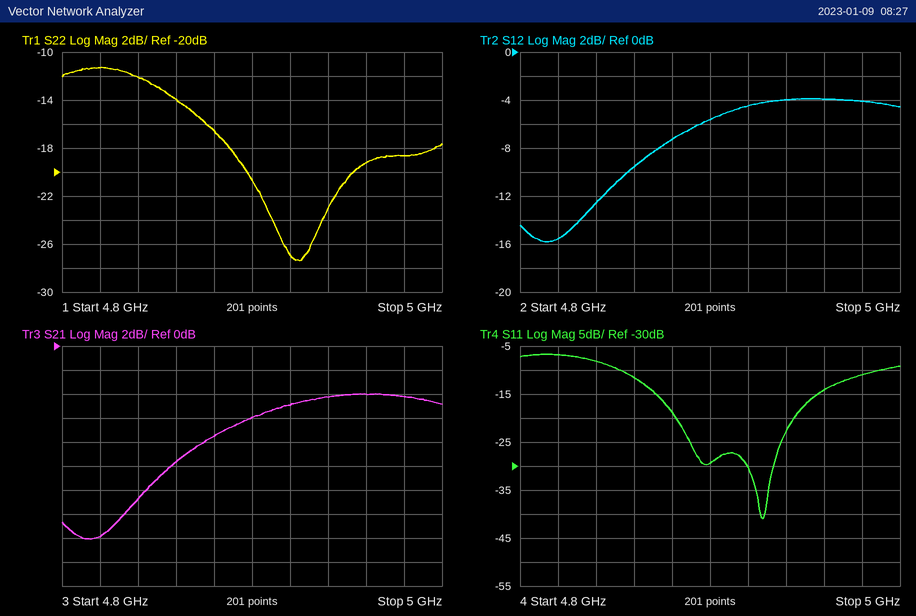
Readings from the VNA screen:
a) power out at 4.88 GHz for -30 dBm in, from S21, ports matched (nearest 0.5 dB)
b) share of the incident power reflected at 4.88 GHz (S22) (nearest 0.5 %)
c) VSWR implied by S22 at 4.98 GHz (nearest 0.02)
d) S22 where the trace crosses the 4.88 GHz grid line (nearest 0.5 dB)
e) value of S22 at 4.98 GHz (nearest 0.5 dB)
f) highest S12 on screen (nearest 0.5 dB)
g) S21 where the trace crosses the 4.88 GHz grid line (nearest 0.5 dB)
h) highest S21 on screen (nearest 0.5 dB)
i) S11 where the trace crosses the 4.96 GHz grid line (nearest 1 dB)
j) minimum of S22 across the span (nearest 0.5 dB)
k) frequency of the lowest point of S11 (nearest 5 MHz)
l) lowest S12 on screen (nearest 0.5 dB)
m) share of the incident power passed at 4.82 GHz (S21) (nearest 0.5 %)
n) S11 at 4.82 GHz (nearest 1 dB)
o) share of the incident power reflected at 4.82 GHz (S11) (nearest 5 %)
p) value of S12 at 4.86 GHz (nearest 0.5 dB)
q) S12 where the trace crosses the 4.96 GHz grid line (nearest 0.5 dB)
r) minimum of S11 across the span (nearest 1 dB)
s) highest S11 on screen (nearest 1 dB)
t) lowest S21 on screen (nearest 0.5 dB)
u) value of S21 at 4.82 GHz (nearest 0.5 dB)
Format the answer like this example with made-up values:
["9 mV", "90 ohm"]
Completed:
["-37.5 dBm", "2.0 %", "1.26", "-16.5 dB", "-18.5 dB", "-4.0 dB", "-7.5 dB", "-4.0 dB", "-14 dB", "-27.5 dB", "4.930 GHz", "-16.0 dB", "2.5 %", "-7 dB", "20 %", "-9.5 dB", "-4.0 dB", "-41 dB", "-7 dB", "-16.0 dB", "-16.0 dB"]
